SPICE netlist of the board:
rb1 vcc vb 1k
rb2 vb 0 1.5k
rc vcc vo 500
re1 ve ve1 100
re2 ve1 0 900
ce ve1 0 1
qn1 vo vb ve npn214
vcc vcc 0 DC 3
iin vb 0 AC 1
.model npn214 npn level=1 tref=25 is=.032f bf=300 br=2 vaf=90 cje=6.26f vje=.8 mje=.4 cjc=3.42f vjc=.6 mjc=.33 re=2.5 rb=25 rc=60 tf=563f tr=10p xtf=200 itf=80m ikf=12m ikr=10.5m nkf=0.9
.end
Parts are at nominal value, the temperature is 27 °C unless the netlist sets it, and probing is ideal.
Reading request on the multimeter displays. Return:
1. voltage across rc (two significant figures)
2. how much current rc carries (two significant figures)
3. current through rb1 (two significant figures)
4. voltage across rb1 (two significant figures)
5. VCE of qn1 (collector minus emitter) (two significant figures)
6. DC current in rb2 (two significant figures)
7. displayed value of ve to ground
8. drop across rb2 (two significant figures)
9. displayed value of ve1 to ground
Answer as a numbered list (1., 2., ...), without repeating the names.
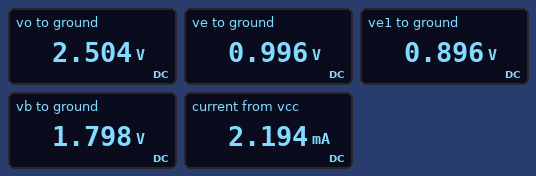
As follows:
1. 500 mV
2. 990 µA
3. 1.2 mA
4. 1.2 V
5. 1.5 V
6. 1.2 mA
7. 0.996 V
8. 1.8 V
9. 0.896 V
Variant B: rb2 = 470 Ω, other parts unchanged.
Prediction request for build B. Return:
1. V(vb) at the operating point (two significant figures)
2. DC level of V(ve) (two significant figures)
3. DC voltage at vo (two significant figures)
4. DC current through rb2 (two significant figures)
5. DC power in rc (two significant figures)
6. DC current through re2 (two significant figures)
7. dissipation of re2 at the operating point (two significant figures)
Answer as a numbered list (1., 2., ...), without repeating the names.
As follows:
1. 960 mV
2. 200 mV
3. 2.9 V
4. 2.0 mA
5. 21 µW
6. 200 µA
7. 37 µW
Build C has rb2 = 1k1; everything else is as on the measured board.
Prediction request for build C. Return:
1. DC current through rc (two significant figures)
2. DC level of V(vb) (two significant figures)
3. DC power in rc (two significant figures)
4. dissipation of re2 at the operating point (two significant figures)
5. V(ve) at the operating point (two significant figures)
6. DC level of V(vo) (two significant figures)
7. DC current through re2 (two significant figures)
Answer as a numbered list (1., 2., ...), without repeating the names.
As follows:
1. 770 µA
2. 1.6 V
3. 300 µW
4. 540 µW
5. 780 mV
6. 2.6 V
7. 780 µA
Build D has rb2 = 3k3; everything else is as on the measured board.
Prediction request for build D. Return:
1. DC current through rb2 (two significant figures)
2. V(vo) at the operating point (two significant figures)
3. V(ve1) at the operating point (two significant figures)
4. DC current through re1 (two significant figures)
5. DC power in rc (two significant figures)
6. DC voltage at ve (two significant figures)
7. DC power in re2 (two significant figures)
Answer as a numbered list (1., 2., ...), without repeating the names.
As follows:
1. 700 µA
2. 2.3 V
3. 1.3 V
4. 1.5 mA
5. 1.1 mW
6. 1.5 V
7. 2.0 mW
